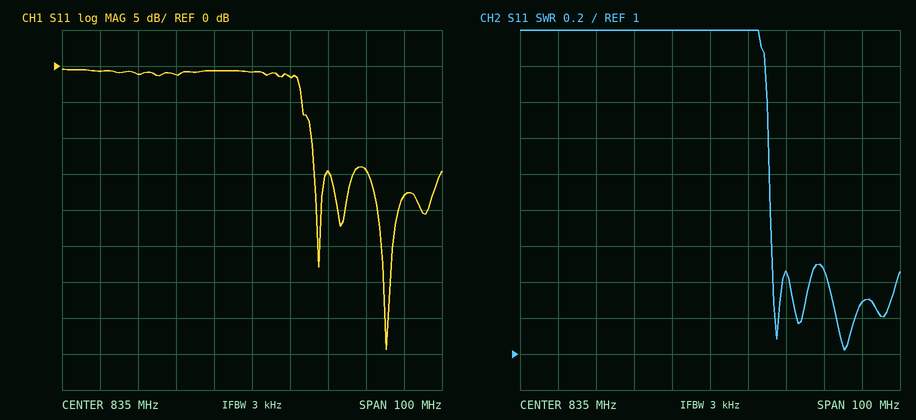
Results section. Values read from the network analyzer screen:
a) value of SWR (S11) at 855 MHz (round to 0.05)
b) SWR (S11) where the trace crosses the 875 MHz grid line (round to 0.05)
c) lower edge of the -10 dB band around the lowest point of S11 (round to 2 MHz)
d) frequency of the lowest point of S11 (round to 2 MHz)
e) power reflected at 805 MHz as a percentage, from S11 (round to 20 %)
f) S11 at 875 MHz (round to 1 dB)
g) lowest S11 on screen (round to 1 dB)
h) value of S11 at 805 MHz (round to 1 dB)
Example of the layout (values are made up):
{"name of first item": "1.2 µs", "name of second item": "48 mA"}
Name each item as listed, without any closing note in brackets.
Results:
{"value of SWR (S11) at 855 MHz": "1.45", "SWR (S11) where the trace crosses the 875 MHz grid line": "1.30", "lower edge of the -10 dB band around the lowest point of S11": "850 MHz", "frequency of the lowest point of S11": "870 MHz", "power reflected at 805 MHz as a percentage, from S11": "80 %", "S11 at 875 MHz": "-18 dB", "lowest S11 on screen": "-39 dB", "value of S11 at 805 MHz": "-1 dB"}
